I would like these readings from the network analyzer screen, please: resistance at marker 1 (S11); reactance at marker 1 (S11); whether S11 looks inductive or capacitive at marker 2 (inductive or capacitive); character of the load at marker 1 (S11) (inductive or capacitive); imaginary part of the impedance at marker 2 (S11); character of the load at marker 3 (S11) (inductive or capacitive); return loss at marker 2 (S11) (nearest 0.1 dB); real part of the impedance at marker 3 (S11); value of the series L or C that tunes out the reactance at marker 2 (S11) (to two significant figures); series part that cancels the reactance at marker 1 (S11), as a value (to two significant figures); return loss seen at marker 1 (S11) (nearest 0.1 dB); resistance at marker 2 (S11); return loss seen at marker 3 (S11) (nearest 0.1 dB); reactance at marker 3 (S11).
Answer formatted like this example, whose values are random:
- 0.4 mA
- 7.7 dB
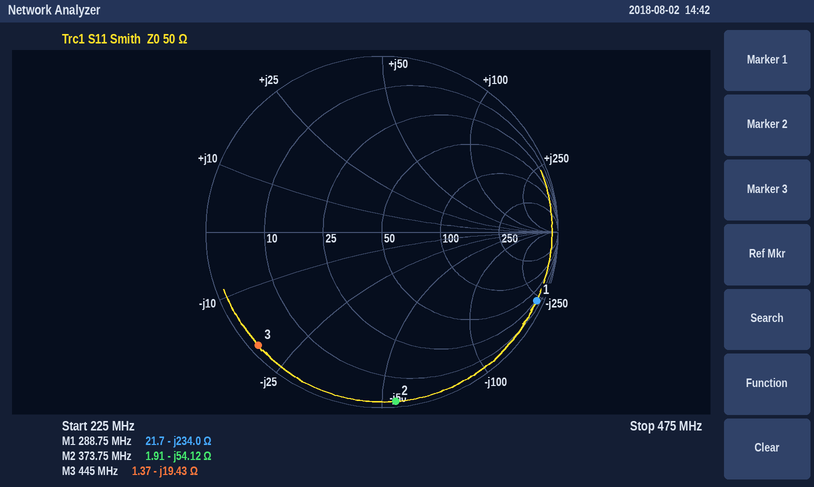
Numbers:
- 21.7 Ω
- -234.0 Ω
- capacitive
- capacitive
- -54.12 Ω
- capacitive
- 0.3 dB
- 1.37 Ω
- 23 nH
- 130 nH
- 0.3 dB
- 1.91 Ω
- 0.4 dB
- -19.43 Ω
